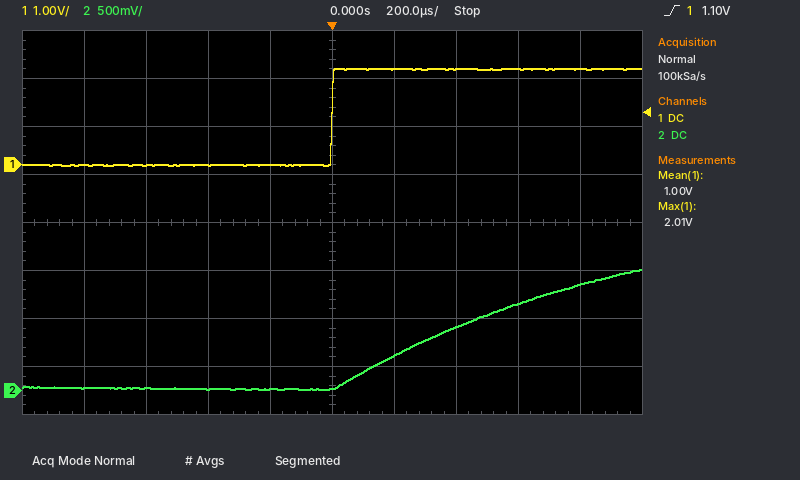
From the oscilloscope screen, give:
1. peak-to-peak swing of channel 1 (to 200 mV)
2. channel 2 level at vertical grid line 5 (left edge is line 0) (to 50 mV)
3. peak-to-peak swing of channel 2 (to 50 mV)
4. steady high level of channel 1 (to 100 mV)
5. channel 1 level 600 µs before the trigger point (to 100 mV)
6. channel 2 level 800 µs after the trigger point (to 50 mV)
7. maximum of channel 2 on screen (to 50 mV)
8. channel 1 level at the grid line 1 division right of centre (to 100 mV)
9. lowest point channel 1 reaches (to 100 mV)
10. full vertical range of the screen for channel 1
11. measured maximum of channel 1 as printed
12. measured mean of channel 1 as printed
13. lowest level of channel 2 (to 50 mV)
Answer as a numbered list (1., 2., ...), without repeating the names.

1. 2.0 V
2. 0 mV
3. 1.25 V
4. 2.0 V
5. 0.0 V
6. 1.10 V
7. 1.25 V
8. 2.0 V
9. 0.0 V
10. 8 V
11. 2.01 V
12. 1.00 V
13. 0 mV
